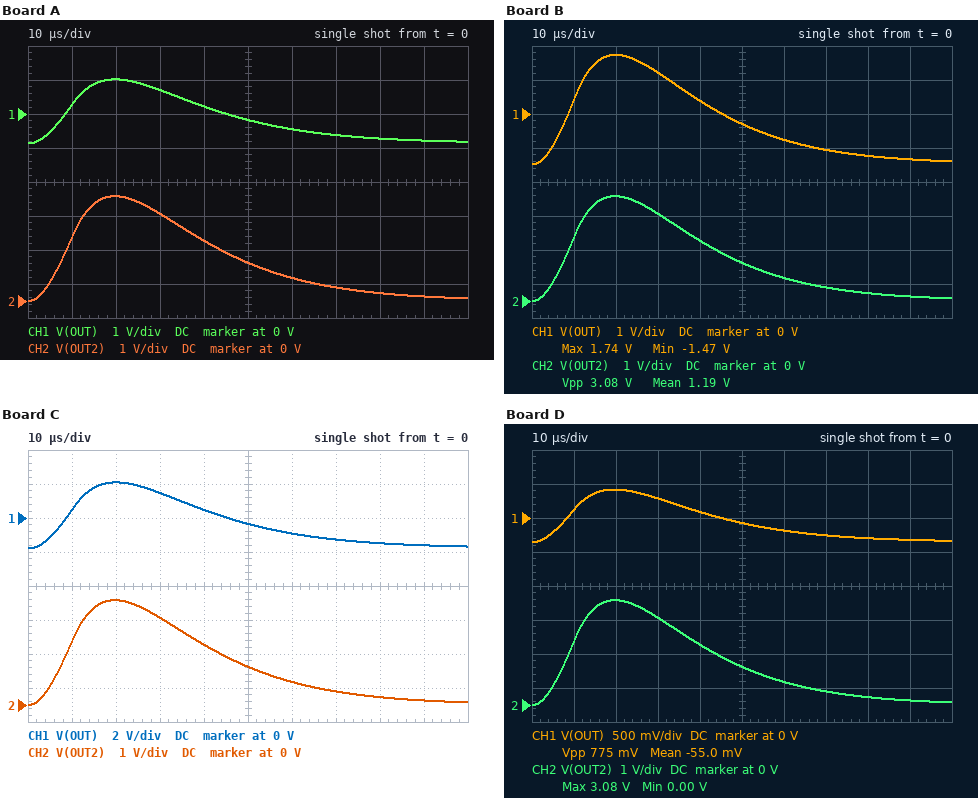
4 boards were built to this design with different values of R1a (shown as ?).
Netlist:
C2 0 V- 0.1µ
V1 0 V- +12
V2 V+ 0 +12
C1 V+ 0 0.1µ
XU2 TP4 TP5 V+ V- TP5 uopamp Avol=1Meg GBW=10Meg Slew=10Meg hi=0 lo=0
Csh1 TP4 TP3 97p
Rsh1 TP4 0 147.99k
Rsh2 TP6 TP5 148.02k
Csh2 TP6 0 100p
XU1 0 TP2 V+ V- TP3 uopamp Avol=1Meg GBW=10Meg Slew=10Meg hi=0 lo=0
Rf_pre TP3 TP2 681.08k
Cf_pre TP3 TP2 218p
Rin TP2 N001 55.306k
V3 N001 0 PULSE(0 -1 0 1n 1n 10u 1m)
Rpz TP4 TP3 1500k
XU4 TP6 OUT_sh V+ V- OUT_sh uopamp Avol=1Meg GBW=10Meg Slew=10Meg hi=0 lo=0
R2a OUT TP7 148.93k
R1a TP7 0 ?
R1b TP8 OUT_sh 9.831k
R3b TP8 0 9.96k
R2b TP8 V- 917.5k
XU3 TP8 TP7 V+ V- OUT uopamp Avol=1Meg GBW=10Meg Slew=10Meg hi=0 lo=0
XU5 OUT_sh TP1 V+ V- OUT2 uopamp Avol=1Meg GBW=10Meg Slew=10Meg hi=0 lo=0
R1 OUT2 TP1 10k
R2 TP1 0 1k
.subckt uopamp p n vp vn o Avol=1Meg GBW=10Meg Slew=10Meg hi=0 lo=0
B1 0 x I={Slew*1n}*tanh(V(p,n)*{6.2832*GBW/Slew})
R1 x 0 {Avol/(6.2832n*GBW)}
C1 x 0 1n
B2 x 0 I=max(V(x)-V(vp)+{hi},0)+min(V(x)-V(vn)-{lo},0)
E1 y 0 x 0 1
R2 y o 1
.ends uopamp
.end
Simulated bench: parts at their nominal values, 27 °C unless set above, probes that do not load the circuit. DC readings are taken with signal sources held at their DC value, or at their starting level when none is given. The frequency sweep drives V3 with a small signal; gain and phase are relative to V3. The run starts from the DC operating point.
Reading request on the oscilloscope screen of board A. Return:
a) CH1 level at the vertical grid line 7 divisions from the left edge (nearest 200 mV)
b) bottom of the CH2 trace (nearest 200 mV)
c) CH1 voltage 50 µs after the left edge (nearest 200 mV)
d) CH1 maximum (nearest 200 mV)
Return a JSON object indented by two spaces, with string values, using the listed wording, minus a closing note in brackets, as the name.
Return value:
{
  "CH1 level at the vertical grid line 7 divisions from the left edge": "-600 mV",
  "bottom of the CH2 trace": "0 V",
  "CH1 voltage 50 µs after the left edge": "-200 mV",
  "CH1 maximum": "1.0 V"
}
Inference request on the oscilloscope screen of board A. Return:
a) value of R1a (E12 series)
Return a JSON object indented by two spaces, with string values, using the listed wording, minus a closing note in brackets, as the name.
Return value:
{
  "value of R1a": "12 kΩ"
}
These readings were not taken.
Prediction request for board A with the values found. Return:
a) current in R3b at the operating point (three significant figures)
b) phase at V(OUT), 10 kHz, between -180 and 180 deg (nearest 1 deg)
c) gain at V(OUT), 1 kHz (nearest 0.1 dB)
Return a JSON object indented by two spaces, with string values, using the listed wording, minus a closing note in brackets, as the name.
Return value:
{
  "current in R3b at the operating point": "6.46 µA",
  "phase at V(OUT), 10 kHz, between -180 and 180 deg": "97 deg",
  "gain at V(OUT), 1 kHz": "17.3 dB"
}
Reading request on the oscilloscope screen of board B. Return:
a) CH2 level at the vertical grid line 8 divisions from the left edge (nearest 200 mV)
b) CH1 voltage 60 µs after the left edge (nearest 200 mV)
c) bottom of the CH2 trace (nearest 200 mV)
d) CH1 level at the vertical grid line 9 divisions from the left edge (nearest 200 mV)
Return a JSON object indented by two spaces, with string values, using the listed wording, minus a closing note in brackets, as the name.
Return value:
{
  "CH2 level at the vertical grid line 8 divisions from the left edge": "200 mV",
  "CH1 voltage 60 µs after the left edge": "-800 mV",
  "bottom of the CH2 trace": "0 V",
  "CH1 level at the vertical grid line 9 divisions from the left edge": "-1.4 V"
}
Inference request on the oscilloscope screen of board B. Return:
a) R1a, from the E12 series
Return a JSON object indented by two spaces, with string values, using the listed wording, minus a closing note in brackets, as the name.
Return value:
{
  "R1a, from the E12 series": "6.8 kΩ"
}
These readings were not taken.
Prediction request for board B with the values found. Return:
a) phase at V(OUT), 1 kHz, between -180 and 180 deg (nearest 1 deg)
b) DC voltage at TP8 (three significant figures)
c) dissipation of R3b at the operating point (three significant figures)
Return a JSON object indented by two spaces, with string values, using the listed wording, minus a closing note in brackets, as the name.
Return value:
{
  "phase at V(OUT), 1 kHz, between -180 and 180 deg": "169 deg",
  "DC voltage at TP8": "-64.4 mV",
  "dissipation of R3b at the operating point": "416 nW"
}
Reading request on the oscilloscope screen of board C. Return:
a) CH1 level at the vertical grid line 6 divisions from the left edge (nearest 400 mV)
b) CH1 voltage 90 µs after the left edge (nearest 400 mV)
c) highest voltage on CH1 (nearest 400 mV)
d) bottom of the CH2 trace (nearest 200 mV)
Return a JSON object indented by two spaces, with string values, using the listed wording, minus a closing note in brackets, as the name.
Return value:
{
  "CH1 level at the vertical grid line 6 divisions from the left edge": "-800 mV",
  "CH1 voltage 90 µs after the left edge": "-1.6 V",
  "highest voltage on CH1": "2.0 V",
  "bottom of the CH2 trace": "0 V"
}
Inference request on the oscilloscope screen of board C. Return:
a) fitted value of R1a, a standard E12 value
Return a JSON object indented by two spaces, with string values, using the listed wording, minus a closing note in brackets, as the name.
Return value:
{
  "fitted value of R1a, a standard E12 value": "5.6 kΩ"
}
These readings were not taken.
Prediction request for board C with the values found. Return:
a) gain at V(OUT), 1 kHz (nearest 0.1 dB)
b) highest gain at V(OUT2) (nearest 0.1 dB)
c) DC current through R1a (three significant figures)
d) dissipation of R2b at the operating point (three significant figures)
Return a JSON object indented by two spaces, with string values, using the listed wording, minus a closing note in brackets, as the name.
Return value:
{
  "gain at V(OUT), 1 kHz": "23.5 dB",
  "highest gain at V(OUT2)": "21.7 dB",
  "DC current through R1a": "11.5 µA",
  "dissipation of R2b at the operating point": "155 µW"
}
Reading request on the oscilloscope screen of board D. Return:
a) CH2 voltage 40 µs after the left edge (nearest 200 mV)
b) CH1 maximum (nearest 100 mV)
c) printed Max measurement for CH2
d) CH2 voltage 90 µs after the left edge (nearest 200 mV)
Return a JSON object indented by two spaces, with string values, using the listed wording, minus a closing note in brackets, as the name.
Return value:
{
  "CH2 voltage 40 µs after the left edge": "1.8 V",
  "CH1 maximum": "400 mV",
  "printed Max measurement for CH2": "3.08 V",
  "CH2 voltage 90 µs after the left edge": "200 mV"
}
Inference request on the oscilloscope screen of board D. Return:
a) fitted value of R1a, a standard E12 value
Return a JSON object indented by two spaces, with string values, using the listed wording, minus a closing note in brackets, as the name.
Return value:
{
  "fitted value of R1a, a standard E12 value": "33 kΩ"
}
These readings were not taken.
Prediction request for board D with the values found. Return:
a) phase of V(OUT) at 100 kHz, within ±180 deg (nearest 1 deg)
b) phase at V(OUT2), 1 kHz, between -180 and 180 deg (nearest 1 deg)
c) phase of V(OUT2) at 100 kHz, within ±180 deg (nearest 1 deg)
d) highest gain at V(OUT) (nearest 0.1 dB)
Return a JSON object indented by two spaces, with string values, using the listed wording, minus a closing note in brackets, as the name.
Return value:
{
  "phase of V(OUT) at 100 kHz, within ±180 deg": "8 deg",
  "phase at V(OUT2), 1 kHz, between -180 and 180 deg": "169 deg",
  "phase of V(OUT2) at 100 kHz, within ±180 deg": "5 deg",
  "highest gain at V(OUT)": "9.7 dB"
}
